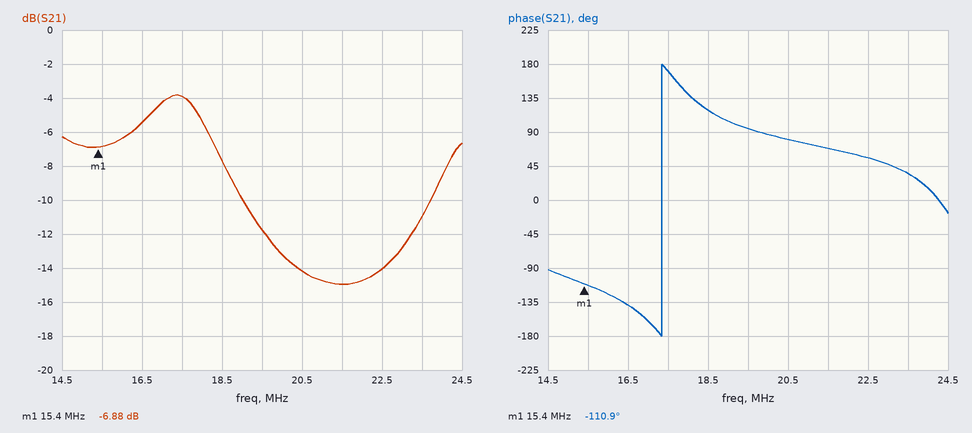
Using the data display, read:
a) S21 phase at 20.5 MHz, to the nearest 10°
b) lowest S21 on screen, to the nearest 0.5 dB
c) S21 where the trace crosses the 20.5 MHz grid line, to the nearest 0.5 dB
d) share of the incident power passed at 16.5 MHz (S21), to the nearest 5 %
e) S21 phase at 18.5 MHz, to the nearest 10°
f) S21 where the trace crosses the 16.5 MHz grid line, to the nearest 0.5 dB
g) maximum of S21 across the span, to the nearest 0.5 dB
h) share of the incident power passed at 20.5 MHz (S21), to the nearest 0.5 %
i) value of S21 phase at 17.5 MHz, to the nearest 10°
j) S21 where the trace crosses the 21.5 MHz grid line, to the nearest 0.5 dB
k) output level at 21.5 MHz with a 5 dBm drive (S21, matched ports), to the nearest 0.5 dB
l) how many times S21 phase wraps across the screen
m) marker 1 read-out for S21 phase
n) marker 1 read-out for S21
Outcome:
80°
-15.0 dB
-14.0 dB
30 %
120°
-5.5 dB
-4.0 dB
4.0 %
170°
-15.0 dB
-10.0 dBm
1
-110.9°
-6.88 dB
